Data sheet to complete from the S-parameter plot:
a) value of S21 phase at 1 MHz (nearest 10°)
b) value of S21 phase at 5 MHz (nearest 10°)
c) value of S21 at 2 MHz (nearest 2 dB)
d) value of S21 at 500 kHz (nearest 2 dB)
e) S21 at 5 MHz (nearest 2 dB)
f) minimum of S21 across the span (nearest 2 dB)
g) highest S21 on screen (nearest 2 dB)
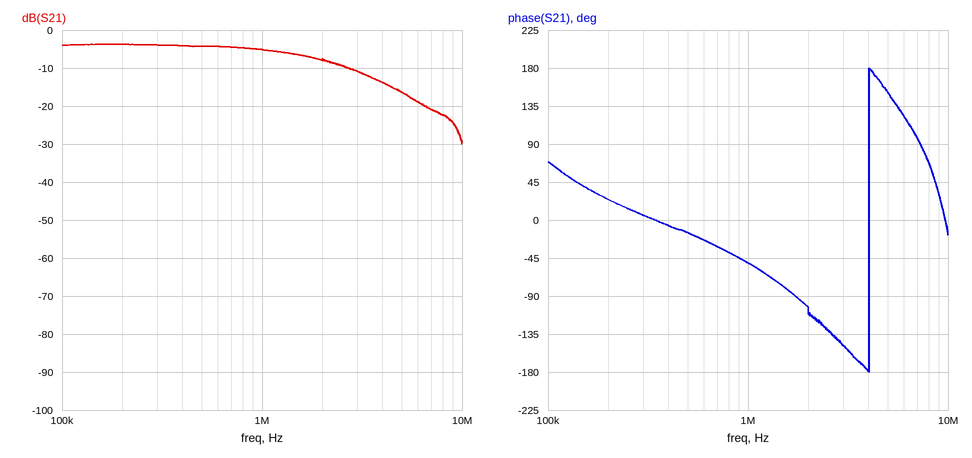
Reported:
-50°
150°
-8 dB
-4 dB
-16 dB
-30 dB
-4 dB
